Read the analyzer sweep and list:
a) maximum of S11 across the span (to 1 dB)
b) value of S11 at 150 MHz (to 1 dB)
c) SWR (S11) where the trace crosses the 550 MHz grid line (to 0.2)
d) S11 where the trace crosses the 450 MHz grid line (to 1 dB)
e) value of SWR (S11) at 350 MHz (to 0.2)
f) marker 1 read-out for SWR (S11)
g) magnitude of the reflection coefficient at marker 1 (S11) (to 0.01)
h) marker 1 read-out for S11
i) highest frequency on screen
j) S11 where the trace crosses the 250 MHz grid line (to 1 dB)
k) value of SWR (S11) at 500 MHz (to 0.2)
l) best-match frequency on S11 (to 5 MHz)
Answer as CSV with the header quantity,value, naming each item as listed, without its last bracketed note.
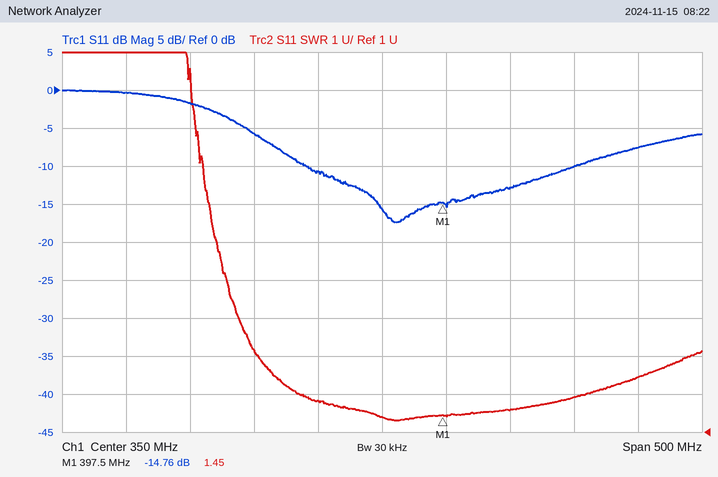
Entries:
quantity,value
maximum of S11 across the span,0 dB
value of S11 at 150 MHz,0 dB
SWR (S11) where the trace crosses the 550 MHz grid line,2.4
S11 where the trace crosses the 450 MHz grid line,-13 dB
value of SWR (S11) at 350 MHz,1.4
marker 1 read-out for SWR,1.45
magnitude of the reflection coefficient at marker 1 (S11),0.18
marker 1 read-out for S11,-14.76 dB
highest frequency on screen,600 MHz
S11 where the trace crosses the 250 MHz grid line,-6 dB
value of SWR (S11) at 500 MHz,2.0
best-match frequency on S11,360 MHz
